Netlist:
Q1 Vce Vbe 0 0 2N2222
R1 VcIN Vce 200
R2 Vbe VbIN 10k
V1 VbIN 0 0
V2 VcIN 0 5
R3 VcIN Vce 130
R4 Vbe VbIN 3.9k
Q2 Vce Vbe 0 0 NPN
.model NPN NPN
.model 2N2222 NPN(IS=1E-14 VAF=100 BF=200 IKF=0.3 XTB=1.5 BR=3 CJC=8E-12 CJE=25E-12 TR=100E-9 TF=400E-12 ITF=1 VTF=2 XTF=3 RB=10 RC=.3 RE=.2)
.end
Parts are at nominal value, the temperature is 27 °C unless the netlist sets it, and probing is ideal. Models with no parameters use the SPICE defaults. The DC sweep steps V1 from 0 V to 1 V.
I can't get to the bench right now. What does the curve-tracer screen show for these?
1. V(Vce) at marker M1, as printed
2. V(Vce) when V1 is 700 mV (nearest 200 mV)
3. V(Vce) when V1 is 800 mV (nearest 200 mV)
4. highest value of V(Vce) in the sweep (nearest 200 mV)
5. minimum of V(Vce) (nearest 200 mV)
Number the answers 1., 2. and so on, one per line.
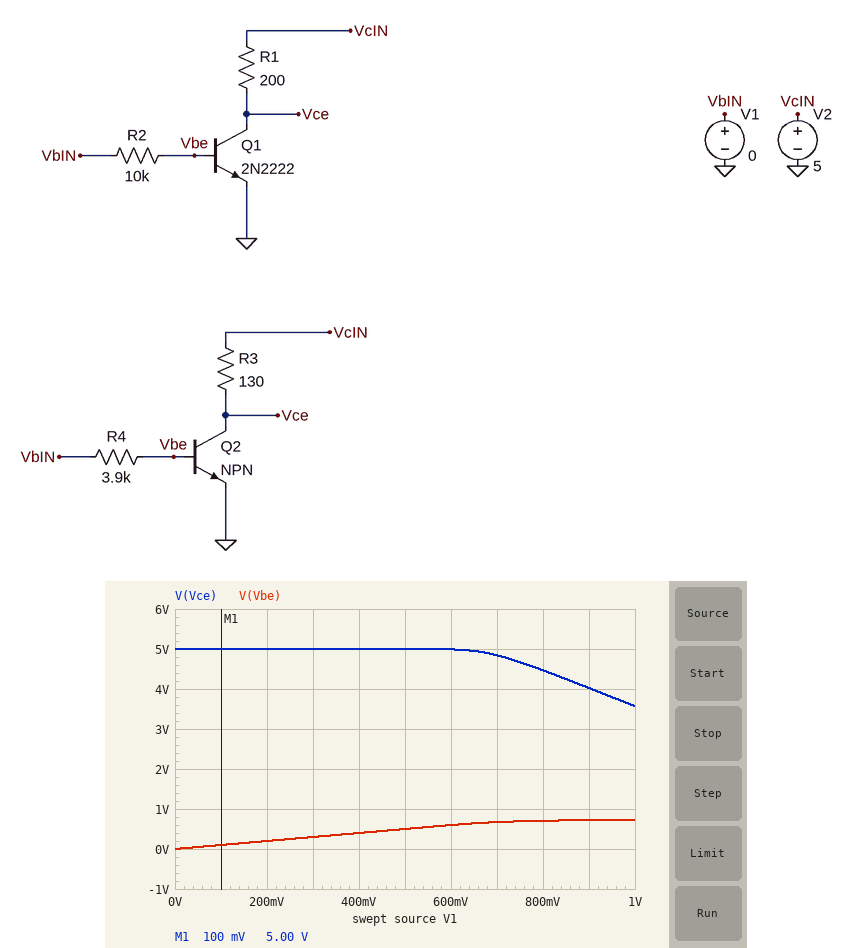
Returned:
1. 5.00 V
2. 4.8 V
3. 4.4 V
4. 5.0 V
5. 3.6 V
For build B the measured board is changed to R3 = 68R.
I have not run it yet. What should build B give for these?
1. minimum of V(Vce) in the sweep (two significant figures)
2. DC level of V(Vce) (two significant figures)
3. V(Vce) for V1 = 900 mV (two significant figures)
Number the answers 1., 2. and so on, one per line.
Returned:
1. 4.1 V
2. 5.0 V
3. 4.4 V
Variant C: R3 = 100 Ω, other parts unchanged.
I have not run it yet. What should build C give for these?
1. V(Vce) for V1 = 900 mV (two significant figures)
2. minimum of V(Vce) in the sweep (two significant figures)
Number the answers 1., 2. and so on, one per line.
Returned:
1. 4.2 V
2. 3.8 V
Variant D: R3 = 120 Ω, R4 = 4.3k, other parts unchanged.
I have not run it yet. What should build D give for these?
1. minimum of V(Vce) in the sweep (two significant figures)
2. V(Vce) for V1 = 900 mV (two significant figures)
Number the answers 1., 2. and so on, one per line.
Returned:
1. 3.7 V
2. 4.1 V
